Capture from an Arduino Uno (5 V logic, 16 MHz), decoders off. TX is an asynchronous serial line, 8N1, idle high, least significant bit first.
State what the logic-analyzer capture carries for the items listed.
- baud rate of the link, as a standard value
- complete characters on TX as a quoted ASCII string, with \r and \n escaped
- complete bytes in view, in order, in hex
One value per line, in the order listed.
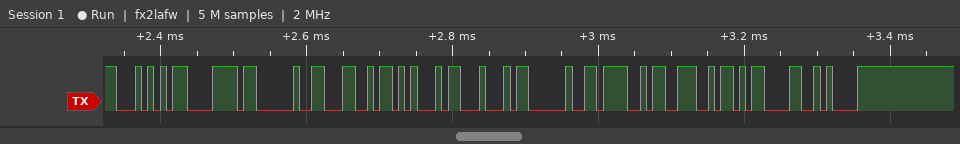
115200 baud
"Tx LED ON\r\n"
0x54 0x78 0x20 0x4C 0x45 0x44 0x20 0x4F 0x4E 0x0D 0x0A
